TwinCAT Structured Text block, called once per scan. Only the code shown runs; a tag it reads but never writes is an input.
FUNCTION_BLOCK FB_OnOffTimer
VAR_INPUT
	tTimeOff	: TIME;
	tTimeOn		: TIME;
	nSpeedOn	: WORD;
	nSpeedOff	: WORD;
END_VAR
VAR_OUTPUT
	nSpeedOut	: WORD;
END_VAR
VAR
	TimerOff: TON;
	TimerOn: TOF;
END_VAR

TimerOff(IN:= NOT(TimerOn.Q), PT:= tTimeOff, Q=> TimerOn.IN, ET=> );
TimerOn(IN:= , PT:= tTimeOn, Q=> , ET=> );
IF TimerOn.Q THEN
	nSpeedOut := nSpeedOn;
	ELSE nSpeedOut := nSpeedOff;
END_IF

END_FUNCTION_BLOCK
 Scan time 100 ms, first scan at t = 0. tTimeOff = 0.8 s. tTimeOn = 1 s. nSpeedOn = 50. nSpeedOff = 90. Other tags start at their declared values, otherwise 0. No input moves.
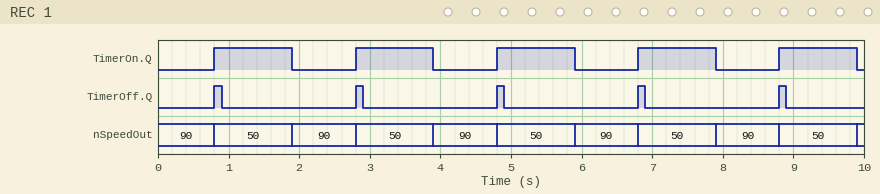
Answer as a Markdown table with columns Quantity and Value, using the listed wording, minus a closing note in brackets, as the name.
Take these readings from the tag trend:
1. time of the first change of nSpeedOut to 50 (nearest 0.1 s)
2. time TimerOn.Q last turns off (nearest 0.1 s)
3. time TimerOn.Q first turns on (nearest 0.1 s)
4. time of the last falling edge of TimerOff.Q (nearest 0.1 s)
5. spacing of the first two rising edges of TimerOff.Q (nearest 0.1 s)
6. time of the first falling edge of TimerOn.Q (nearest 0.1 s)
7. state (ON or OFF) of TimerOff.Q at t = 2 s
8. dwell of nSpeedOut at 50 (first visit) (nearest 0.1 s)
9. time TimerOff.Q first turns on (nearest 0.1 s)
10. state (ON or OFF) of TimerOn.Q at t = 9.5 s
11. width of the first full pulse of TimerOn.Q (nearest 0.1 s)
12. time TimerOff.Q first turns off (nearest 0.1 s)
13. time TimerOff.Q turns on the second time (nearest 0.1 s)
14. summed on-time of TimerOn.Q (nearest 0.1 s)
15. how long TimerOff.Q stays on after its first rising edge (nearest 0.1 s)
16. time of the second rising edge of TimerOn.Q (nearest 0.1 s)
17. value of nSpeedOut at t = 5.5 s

| Quantity | Value |
|---|---|
| time of the first change of nSpeedOut to 50 | 0.8 s |
| time TimerOn.Q last turns off | 9.9 s |
| time TimerOn.Q first turns on | 0.8 s |
| time of the last falling edge of TimerOff.Q | 8.9 s |
| spacing of the first two rising edges of TimerOff.Q | 2.0 s |
| time of the first falling edge of TimerOn.Q | 1.9 s |
| state (ON or OFF) of TimerOff.Q at t = 2 s | OFF |
| dwell of nSpeedOut at 50 (first visit) | 1.1 s |
| time TimerOff.Q first turns on | 0.8 s |
| state (ON or OFF) of TimerOn.Q at t = 9.5 s | ON |
| width of the first full pulse of TimerOn.Q | 1.1 s |
| time TimerOff.Q first turns off | 0.9 s |
| time TimerOff.Q turns on the second time | 2.8 s |
| summed on-time of TimerOn.Q | 5.5 s |
| how long TimerOff.Q stays on after its first rising edge | 0.1 s |
| time of the second rising edge of TimerOn.Q | 2.8 s |
| value of nSpeedOut at t = 5.5 s | 50 |
